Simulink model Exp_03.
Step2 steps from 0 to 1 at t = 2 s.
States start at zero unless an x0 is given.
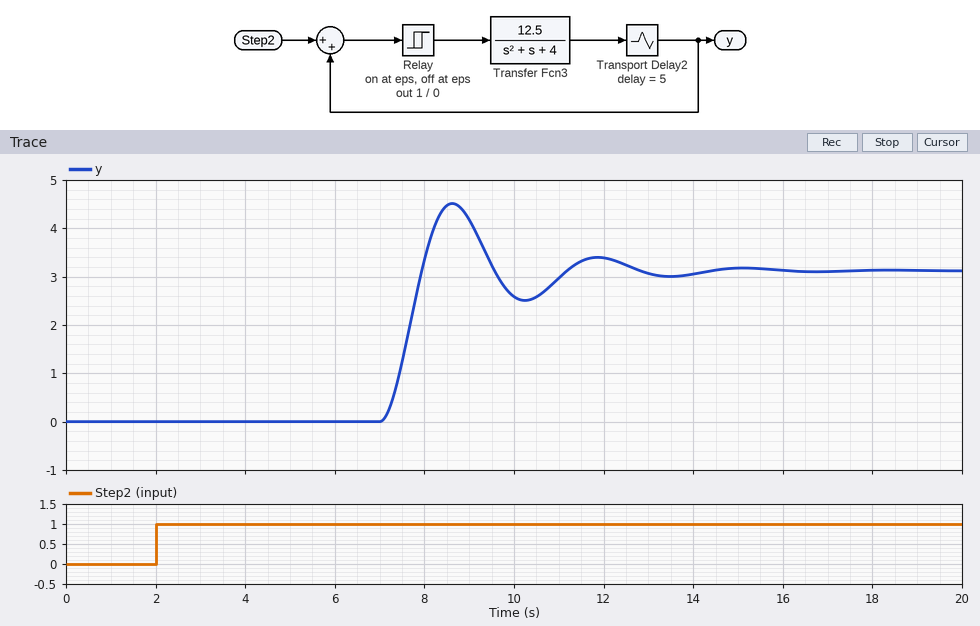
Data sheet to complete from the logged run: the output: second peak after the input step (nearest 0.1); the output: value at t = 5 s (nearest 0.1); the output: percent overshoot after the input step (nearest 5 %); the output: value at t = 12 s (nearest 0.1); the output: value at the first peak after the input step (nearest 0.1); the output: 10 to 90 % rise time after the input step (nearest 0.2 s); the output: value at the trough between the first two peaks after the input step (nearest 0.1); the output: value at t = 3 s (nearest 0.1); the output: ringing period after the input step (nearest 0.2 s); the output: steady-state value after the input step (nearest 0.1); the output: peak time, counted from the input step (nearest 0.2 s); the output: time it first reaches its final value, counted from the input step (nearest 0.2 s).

3.4
0.0
45 %
3.4
4.5
0.6 s
2.5
0.0
3.2 s
3.1
6.6 s
6.0 s
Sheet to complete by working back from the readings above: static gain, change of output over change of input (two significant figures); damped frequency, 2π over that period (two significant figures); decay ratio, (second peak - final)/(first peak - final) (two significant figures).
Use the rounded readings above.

3.1
2.0 rad/s
0.21
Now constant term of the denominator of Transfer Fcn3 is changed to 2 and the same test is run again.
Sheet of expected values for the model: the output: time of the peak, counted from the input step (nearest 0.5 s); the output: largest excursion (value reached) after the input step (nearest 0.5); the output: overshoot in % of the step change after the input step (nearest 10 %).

7.5 s
8.0
30 %
